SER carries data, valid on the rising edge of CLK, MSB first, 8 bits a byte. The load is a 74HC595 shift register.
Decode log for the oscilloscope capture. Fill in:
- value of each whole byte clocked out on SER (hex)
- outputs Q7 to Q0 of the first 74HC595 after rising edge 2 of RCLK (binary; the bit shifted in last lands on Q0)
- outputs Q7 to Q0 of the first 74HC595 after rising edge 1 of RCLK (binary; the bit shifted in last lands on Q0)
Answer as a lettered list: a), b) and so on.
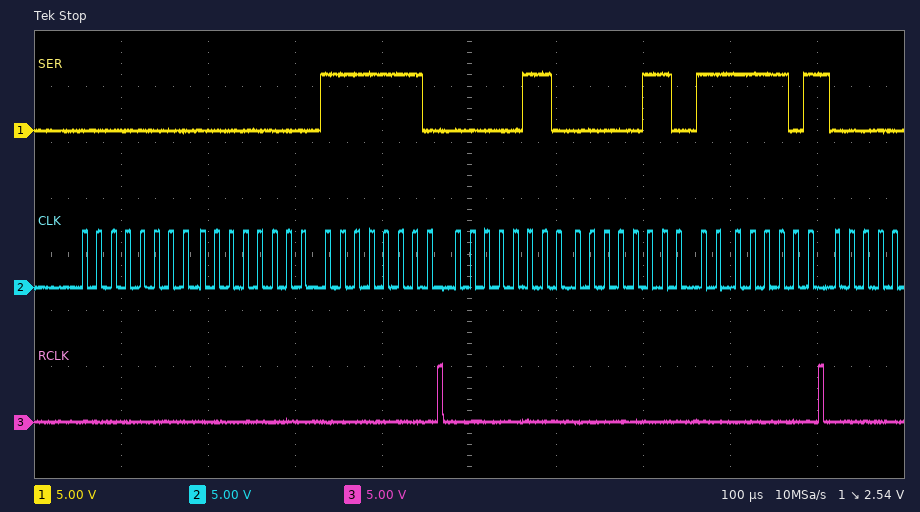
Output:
a) 0x00 0x00 0xFE 0x06 0x06 0xFD
b) 11111101
c) 11111110
